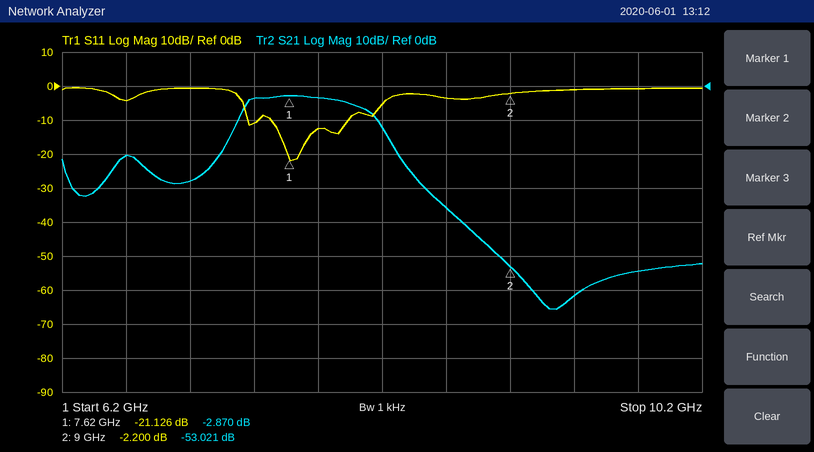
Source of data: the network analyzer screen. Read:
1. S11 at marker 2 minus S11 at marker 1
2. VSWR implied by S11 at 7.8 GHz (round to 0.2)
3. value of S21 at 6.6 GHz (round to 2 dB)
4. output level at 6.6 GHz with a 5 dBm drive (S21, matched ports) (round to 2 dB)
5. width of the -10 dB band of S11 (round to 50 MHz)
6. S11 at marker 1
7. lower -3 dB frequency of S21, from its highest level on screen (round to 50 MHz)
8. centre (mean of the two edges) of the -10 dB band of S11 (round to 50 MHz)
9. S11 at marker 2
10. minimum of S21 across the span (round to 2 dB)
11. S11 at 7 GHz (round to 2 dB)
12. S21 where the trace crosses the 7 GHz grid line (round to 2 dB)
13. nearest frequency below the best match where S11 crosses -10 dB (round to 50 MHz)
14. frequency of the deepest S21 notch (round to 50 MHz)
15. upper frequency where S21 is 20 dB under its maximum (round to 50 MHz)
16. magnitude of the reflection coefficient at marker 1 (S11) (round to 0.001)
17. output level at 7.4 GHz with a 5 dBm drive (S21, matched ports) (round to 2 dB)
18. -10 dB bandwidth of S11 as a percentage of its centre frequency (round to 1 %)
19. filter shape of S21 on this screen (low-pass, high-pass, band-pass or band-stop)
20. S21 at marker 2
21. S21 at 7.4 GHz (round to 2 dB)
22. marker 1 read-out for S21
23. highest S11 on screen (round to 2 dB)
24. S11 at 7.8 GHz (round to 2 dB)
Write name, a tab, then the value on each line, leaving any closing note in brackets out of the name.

S11 at marker 2 minus S11 at marker 1	18.926 dB
VSWR implied by S11 at 7.8 GHz	1.6
value of S21 at 6.6 GHz	-20 dB
output level at 6.6 GHz with a 5 dBm drive (S21, matched ports)	-16 dBm
width of the -10 dB band of S11	500 MHz
S11 at marker 1	-21.126 dB
lower -3 dB frequency of S21, from its highest level on screen	7.35 GHz
centre (mean of the two edges) of the -10 dB band of S11	7.75 GHz
S11 at marker 2	-2.200 dB
minimum of S21 across the span	-66 dB
S11 at 7 GHz	0 dB
S21 where the trace crosses the 7 GHz grid line	-28 dB
nearest frequency below the best match where S11 crosses -10 dB	7.50 GHz
frequency of the deepest S21 notch	9.30 GHz
upper frequency where S21 is 20 dB under its maximum	8.35 GHz
magnitude of the reflection coefficient at marker 1 (S11)	0.088
output level at 7.4 GHz with a 5 dBm drive (S21, matched ports)	2 dBm
-10 dB bandwidth of S11 as a percentage of its centre frequency	6 %
filter shape of S21 on this screen	band-pass
S21 at marker 2	-53.021 dB
S21 at 7.4 GHz	-4 dB
marker 1 read-out for S21	-2.870 dB
highest S11 on screen	0 dB
S11 at 7.8 GHz	-12 dB
